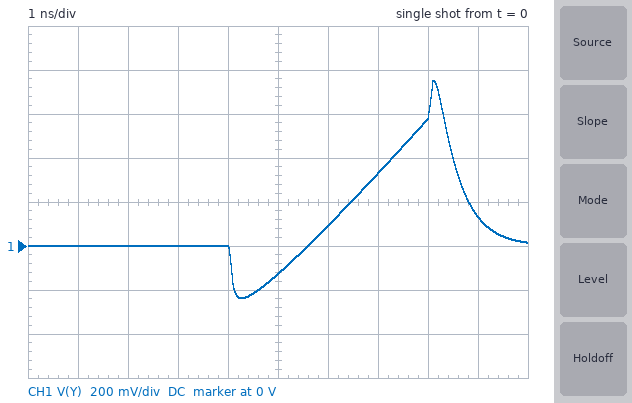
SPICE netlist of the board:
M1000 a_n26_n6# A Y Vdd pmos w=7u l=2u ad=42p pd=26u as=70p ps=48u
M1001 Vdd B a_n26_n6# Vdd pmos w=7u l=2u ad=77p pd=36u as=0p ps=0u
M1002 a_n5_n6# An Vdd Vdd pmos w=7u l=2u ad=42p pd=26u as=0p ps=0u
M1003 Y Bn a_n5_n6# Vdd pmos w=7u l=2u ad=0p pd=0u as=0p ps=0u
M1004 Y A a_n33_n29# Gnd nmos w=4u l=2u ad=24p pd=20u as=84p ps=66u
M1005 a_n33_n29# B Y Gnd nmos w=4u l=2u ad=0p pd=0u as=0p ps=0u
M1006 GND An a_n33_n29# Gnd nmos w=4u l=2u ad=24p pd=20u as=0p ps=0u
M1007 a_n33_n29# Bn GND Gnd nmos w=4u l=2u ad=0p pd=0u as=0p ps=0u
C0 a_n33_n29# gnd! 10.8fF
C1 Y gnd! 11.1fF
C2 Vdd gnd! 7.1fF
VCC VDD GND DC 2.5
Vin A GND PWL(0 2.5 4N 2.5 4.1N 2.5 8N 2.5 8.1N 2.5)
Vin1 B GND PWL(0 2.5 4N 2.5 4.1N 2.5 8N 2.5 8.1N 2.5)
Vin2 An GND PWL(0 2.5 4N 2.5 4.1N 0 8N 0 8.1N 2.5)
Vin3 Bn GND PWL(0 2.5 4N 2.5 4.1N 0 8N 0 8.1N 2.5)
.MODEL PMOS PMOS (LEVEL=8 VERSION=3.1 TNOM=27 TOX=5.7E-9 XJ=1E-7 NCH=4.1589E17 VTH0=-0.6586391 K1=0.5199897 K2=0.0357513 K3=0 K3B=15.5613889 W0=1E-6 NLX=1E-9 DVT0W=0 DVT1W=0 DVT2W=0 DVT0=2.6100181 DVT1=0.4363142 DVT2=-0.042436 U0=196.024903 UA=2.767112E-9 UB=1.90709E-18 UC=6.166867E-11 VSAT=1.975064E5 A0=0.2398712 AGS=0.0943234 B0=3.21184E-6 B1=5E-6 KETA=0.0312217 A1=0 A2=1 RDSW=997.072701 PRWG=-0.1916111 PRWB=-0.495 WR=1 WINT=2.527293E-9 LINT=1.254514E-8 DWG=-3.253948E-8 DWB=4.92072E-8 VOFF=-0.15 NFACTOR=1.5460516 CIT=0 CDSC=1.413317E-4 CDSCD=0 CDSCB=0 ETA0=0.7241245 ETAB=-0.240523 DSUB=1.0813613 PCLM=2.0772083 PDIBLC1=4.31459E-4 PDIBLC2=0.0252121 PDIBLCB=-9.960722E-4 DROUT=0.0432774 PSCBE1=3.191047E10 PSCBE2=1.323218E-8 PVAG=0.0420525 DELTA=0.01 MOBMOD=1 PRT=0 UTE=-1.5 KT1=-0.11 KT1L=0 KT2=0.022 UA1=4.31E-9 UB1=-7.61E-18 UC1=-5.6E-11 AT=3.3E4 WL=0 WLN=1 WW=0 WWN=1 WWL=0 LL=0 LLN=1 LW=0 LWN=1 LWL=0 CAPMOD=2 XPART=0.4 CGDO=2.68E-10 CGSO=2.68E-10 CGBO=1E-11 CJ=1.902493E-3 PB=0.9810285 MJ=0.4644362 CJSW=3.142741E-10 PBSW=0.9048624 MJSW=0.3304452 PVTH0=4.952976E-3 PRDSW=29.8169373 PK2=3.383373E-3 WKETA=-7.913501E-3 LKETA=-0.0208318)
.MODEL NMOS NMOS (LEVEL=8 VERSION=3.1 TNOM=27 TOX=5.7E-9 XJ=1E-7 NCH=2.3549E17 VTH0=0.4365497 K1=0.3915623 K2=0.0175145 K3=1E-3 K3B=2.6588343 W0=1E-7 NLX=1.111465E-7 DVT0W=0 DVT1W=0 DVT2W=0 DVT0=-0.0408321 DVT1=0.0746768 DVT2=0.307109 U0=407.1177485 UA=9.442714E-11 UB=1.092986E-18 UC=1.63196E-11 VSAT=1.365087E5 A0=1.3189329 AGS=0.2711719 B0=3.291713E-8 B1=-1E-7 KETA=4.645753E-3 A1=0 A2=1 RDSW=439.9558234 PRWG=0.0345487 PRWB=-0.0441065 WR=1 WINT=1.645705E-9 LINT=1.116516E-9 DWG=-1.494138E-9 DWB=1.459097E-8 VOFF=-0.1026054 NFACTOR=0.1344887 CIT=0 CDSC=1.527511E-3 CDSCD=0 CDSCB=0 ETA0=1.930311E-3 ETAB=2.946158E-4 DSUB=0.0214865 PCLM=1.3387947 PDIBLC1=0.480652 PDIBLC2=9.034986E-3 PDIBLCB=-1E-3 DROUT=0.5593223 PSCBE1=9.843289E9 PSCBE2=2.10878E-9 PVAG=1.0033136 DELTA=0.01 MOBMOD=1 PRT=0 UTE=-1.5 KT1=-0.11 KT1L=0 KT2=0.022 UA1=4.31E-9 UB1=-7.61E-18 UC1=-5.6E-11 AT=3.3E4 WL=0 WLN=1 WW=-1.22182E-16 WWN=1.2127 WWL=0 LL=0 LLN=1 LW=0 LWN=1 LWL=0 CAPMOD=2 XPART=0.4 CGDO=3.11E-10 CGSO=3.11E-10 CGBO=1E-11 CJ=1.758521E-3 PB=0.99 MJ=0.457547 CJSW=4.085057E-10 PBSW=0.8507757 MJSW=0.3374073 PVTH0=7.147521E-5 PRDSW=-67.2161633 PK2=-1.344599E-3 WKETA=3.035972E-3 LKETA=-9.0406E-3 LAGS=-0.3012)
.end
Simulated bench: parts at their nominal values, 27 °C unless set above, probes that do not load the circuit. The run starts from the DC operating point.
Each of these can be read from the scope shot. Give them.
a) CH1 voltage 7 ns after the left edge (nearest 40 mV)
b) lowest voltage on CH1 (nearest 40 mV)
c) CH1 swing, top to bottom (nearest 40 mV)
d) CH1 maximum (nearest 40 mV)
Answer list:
320 mV
-240 mV
1.00 V
760 mV
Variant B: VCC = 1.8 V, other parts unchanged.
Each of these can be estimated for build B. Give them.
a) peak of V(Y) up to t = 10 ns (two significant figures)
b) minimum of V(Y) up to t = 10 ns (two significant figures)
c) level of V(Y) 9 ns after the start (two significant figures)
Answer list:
270 mV
-230 mV
52 mV
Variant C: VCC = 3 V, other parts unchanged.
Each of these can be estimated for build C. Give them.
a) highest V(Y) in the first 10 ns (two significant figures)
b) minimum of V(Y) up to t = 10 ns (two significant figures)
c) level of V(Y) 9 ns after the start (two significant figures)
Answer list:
1.2 V
-240 mV
240 mV
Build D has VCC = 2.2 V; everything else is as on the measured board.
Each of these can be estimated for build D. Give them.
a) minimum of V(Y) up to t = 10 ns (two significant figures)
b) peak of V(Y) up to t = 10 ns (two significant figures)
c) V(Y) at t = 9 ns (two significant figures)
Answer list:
-240 mV
520 mV
92 mV
